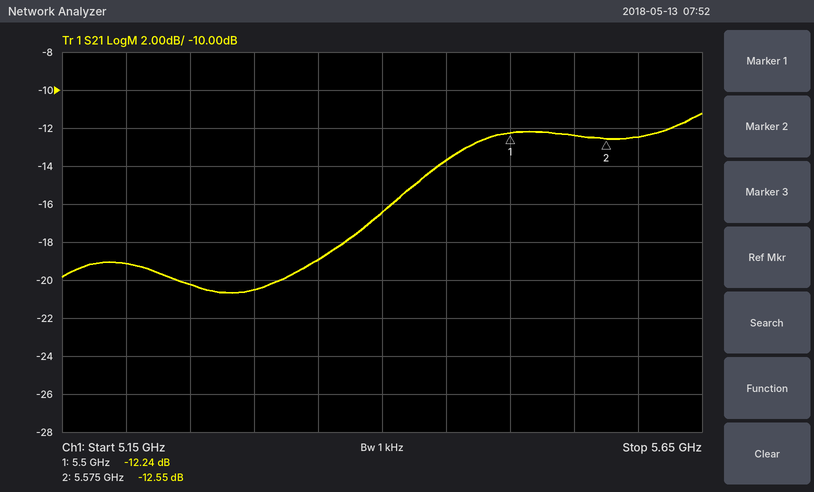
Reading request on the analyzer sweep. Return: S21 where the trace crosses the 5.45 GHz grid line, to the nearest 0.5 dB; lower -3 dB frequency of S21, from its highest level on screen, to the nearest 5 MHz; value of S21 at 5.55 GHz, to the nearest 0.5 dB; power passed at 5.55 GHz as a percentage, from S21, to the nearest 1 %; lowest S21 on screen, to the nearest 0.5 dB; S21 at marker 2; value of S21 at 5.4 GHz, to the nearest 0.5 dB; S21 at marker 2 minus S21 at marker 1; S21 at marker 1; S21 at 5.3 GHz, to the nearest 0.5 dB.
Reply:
-13.5 dB
5.440 GHz
-12.5 dB
6 %
-20.5 dB
-12.55 dB
-16.5 dB
-0.31 dB
-12.24 dB
-20.5 dB
